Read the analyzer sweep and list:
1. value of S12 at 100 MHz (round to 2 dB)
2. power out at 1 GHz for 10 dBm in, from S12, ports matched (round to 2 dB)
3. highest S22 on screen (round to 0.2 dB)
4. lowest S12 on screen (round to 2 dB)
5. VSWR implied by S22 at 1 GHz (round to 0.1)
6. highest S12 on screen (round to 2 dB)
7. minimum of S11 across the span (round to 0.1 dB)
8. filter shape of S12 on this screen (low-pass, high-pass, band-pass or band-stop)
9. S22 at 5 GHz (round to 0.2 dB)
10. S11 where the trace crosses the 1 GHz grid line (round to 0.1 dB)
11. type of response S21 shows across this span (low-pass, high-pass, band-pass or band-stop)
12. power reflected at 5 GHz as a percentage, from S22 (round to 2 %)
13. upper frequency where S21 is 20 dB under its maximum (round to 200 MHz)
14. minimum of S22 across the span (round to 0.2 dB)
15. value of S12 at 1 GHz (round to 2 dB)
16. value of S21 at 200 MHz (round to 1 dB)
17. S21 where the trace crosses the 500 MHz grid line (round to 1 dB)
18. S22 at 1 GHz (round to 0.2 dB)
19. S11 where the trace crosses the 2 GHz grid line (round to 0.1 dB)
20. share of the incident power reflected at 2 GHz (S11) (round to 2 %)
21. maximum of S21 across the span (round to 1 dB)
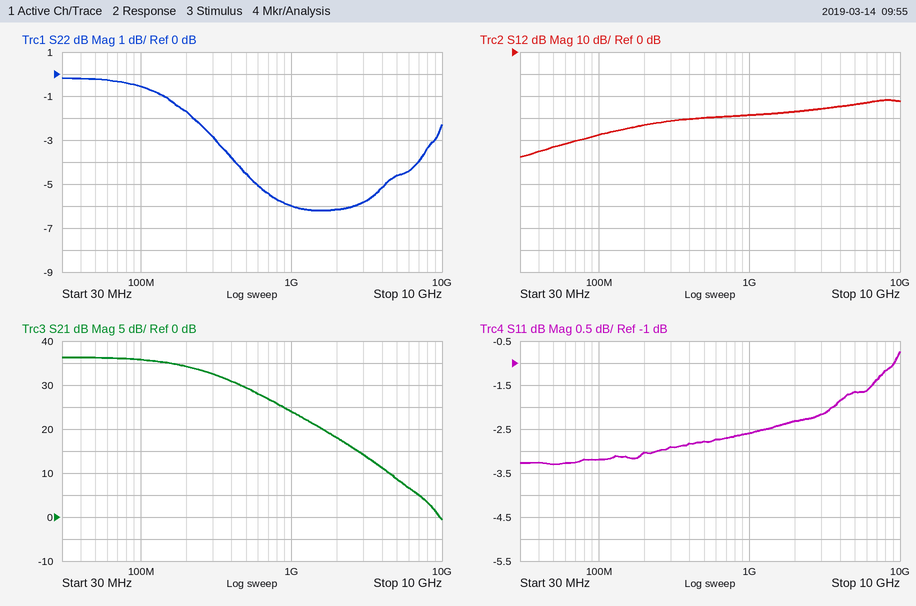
-38 dB
-18 dBm
-0.2 dB
-48 dB
3.0
-22 dB
-3.3 dB
high-pass
-4.6 dB
-2.6 dB
low-pass
34 %
2.4 GHz
-6.2 dB
-28 dB
34 dB
29 dB
-6.0 dB
-2.3 dB
58 %
36 dB
